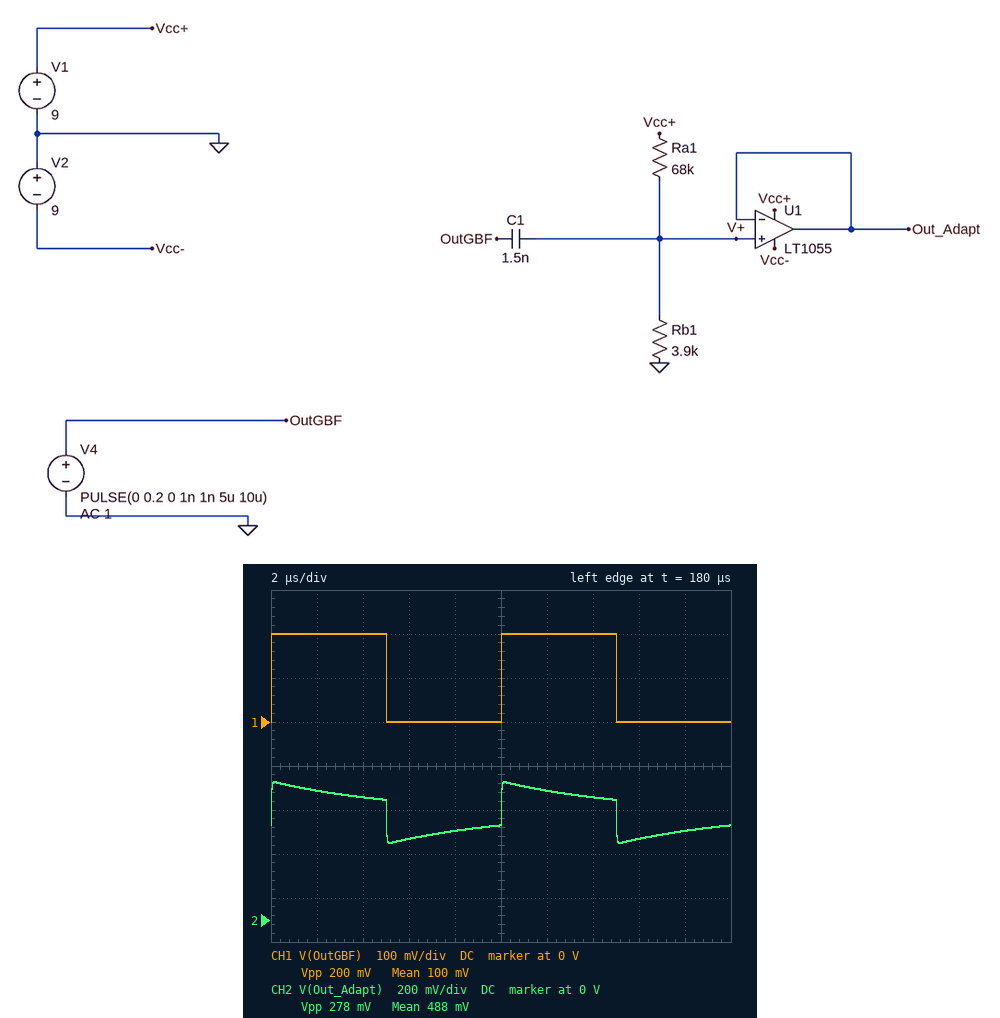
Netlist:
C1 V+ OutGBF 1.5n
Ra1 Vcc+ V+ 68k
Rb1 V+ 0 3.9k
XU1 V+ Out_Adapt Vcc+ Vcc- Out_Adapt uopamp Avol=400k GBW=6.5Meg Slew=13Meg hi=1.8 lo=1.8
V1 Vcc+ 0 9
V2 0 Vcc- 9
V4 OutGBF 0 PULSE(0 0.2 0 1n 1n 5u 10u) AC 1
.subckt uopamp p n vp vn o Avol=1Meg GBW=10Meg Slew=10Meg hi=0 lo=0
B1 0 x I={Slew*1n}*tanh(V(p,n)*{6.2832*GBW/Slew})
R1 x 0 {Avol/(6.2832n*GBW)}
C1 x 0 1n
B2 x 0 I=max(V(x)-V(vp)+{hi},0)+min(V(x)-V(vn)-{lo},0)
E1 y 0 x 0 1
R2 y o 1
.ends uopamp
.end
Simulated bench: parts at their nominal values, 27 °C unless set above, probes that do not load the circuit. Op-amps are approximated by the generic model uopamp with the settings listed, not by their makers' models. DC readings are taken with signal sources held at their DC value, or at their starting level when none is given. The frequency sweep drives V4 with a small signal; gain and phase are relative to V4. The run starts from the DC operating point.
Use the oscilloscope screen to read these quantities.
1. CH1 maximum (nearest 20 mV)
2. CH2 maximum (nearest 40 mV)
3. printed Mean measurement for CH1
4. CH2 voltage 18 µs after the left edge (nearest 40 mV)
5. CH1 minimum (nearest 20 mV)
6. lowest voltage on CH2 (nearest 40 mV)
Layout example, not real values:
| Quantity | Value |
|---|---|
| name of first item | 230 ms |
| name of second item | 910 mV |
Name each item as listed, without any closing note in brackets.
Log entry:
| Quantity | Value |
|---|---|
| CH1 maximum | 200 mV |
| CH2 maximum | 640 mV |
| printed Mean measurement for CH1 | 100 mV |
| CH2 voltage 18 µs after the left edge | 400 mV |
| CH1 minimum | 0 V |
| lowest voltage on CH2 | 360 mV |
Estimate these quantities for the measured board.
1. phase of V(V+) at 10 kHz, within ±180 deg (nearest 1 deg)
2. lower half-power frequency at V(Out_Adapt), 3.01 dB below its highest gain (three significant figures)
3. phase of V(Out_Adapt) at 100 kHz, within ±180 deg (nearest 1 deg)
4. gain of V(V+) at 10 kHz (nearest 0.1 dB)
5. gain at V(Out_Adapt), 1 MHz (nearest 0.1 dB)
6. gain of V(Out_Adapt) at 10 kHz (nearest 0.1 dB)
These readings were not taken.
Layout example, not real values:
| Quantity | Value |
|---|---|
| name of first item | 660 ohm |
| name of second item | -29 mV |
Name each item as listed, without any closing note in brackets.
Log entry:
| Quantity | Value |
|---|---|
| phase of V(V+) at 10 kHz, within ±180 deg | 71 deg |
| lower half-power frequency at V(Out_Adapt), 3.01 dB below its highest gain | 28.5 kHz |
| phase of V(Out_Adapt) at 100 kHz, within ±180 deg | 15 deg |
| gain of V(V+) at 10 kHz | -9.7 dB |
| gain at V(Out_Adapt), 1 MHz | -0.1 dB |
| gain of V(Out_Adapt) at 10 kHz | -9.7 dB |
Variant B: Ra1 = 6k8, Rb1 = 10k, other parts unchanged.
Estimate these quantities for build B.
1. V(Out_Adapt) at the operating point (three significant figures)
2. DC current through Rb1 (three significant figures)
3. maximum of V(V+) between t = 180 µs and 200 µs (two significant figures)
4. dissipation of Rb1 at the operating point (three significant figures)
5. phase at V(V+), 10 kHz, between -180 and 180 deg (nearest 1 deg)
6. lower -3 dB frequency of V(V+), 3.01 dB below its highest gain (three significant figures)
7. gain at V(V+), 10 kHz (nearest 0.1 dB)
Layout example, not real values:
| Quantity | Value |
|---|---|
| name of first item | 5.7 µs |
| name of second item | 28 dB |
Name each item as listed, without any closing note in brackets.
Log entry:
| Quantity | Value |
|---|---|
| V(Out_Adapt) at the operating point | 5.36 V |
| DC current through Rb1 | 536 µA |
| maximum of V(V+) between t = 180 µs and 200 µs | 5.5 V |
| dissipation of Rb1 at the operating point | 2.87 mW |
| phase at V(V+), 10 kHz, between -180 and 180 deg | 69 deg |
| lower -3 dB frequency of V(V+), 3.01 dB below its highest gain | 26.2 kHz |
| gain at V(V+), 10 kHz | -9.0 dB |
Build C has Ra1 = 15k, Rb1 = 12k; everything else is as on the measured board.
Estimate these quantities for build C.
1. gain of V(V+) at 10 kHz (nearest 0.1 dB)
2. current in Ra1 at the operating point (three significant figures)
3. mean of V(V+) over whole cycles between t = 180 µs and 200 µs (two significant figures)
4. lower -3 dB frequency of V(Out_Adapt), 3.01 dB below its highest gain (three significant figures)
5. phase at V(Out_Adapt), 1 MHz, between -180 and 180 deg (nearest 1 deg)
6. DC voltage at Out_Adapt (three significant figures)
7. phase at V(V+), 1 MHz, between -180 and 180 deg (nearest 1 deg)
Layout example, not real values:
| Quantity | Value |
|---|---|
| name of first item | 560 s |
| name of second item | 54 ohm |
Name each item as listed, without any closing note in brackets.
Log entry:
| Quantity | Value |
|---|---|
| gain of V(V+) at 10 kHz | -5.5 dB |
| current in Ra1 at the operating point | 333 µA |
| mean of V(V+) over whole cycles between t = 180 µs and 200 µs | 4.0 V |
| lower -3 dB frequency of V(Out_Adapt), 3.01 dB below its highest gain | 15.8 kHz |
| phase at V(Out_Adapt), 1 MHz, between -180 and 180 deg | -8 deg |
| DC voltage at Out_Adapt | 4.00 V |
| phase at V(V+), 1 MHz, between -180 and 180 deg | 1 deg |
